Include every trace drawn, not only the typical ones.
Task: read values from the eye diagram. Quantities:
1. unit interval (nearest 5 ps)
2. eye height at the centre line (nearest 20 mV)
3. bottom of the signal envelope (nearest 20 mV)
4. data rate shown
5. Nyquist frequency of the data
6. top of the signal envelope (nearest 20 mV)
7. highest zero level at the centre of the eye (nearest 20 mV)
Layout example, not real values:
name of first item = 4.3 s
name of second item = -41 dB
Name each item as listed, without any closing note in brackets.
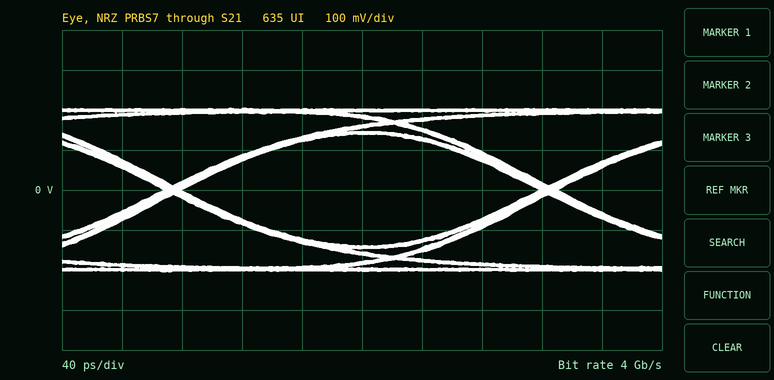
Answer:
unit interval = 250 ps
eye height at the centre line = 280 mV
bottom of the signal envelope = -200 mV
data rate shown = 4 Gb/s
Nyquist frequency of the data = 2 GHz
top of the signal envelope = 200 mV
highest zero level at the centre of the eye = -140 mV
